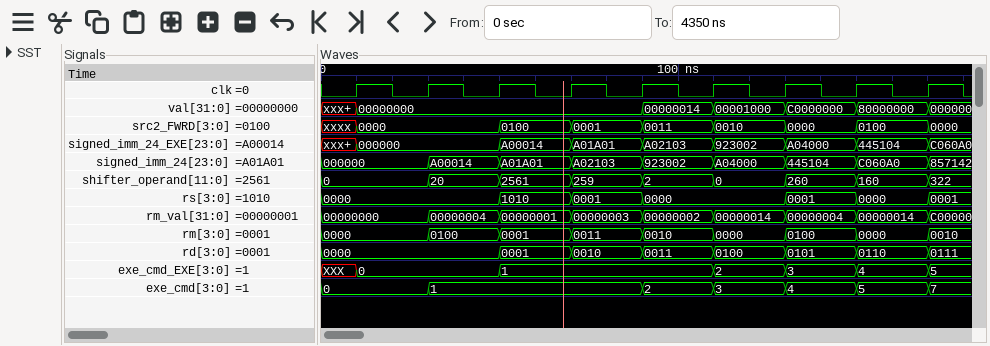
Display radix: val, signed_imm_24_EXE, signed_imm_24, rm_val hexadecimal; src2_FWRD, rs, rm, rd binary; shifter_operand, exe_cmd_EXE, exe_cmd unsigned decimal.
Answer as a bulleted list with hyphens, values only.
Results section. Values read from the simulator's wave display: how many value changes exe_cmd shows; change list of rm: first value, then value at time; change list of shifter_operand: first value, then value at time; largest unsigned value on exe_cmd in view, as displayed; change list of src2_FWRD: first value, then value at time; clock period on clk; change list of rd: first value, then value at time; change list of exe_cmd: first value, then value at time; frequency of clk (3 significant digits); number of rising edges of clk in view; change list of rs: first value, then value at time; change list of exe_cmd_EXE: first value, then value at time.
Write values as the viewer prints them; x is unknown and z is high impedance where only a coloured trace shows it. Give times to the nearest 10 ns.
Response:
- 6
- 0000, 0100 at 30 ns, 0001 at 50 ns, 0011 at 70 ns, 0010 at 90 ns, 0000 at 110 ns, 0100 at 130 ns, 0000 at 150 ns, 0010 at 170 ns
- 0, 20 at 30 ns, 2561 at 50 ns, 259 at 70 ns, 2 at 90 ns, 0 at 110 ns, 260 at 130 ns, 160 at 150 ns, 322 at 170 ns
- 7
- xxxx, 0000 at 10 ns, 0100 at 50 ns, 0001 at 70 ns, 0011 at 90 ns, 0010 at 110 ns, 0000 at 130 ns, 0100 at 150 ns, 0000 at 170 ns
- 20 ns
- 0000, 0001 at 50 ns, 0010 at 70 ns, 0011 at 90 ns, 0100 at 110 ns, 0101 at 130 ns, 0110 at 150 ns, 0111 at 170 ns
- 0, 1 at 30 ns, 2 at 90 ns, 3 at 110 ns, 4 at 130 ns, 5 at 150 ns, 7 at 170 ns
- 50.0 MHz
- 9
- 0000, 1010 at 50 ns, 0001 at 70 ns, 0000 at 90 ns, 0001 at 130 ns, 0000 at 150 ns, 0001 at 170 ns
- XXX, 0 at 10 ns, 1 at 50 ns, 2 at 110 ns, 3 at 130 ns, 4 at 150 ns, 5 at 170 ns
